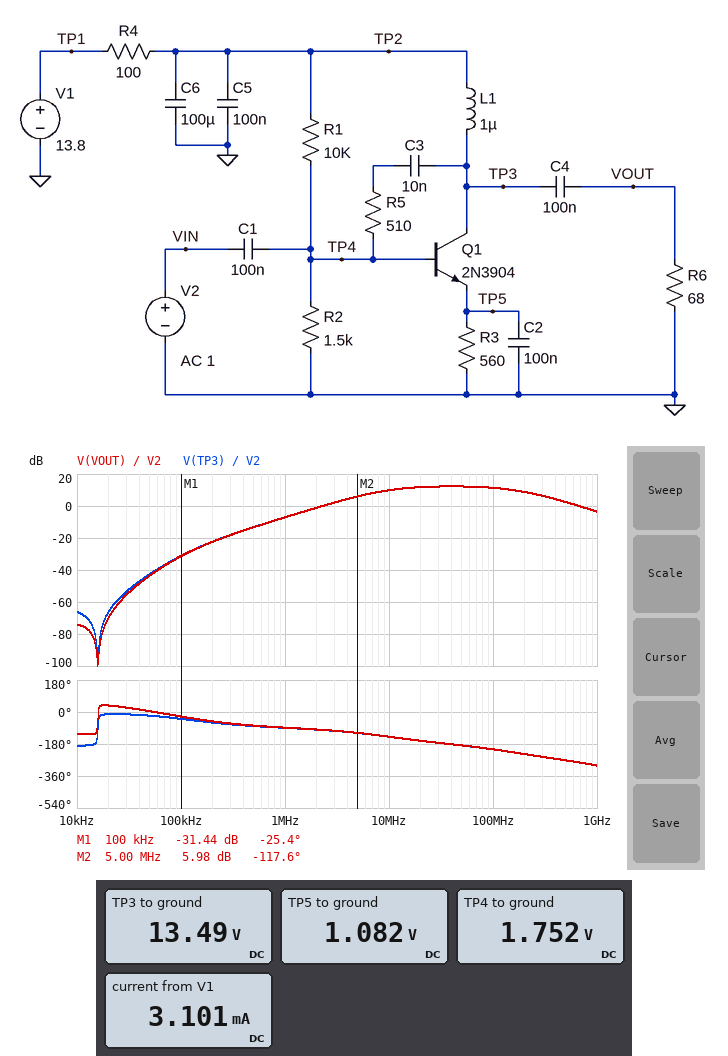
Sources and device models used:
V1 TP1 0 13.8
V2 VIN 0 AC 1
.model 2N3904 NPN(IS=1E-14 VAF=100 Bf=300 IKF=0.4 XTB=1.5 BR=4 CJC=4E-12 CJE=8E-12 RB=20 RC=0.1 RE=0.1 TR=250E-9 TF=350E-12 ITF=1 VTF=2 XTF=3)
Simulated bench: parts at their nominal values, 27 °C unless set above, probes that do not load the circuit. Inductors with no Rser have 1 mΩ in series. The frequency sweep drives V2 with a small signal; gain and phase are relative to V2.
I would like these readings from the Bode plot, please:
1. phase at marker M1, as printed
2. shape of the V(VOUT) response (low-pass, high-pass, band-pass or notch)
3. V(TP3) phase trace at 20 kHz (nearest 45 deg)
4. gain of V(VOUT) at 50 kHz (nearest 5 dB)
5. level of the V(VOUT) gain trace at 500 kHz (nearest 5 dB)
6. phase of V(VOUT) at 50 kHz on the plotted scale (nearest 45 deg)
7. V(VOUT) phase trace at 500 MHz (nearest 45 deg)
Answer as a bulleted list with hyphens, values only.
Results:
- -25.4 deg
- band-pass
- 0 deg
- -45 dB
- -15 dB
- 0 deg
- -270 deg
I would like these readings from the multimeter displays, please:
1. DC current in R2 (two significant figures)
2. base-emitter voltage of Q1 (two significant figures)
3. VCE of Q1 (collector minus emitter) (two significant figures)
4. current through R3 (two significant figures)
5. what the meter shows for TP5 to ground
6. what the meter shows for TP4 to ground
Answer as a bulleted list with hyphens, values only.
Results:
- 1.2 mA
- 670 mV
- 12 V
- 1.9 mA
- 1.082 V
- 1.752 V
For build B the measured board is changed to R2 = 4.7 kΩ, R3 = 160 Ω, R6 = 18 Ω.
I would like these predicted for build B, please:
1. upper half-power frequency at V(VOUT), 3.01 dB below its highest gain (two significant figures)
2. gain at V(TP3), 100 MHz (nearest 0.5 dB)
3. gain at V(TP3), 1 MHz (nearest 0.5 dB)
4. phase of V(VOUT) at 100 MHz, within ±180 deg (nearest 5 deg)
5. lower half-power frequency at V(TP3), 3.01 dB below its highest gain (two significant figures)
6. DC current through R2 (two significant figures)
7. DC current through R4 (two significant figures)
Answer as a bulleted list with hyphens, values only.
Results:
- 37 MHz
- 10.0 dB
- 8.5 dB
- 110 deg
- 2.6 MHz
- 770 µA
- 19 mA
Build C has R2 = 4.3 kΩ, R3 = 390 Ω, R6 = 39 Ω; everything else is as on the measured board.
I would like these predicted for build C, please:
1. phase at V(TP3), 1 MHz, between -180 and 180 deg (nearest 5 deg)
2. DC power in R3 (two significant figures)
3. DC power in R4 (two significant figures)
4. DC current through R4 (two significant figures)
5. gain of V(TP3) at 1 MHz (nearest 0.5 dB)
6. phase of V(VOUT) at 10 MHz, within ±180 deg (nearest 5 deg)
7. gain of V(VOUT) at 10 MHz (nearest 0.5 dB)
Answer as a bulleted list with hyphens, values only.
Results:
- -75 deg
- 25 mW
- 7.8 mW
- 8.8 mA
- 4.0 dB
- -155 deg
- 19.0 dB
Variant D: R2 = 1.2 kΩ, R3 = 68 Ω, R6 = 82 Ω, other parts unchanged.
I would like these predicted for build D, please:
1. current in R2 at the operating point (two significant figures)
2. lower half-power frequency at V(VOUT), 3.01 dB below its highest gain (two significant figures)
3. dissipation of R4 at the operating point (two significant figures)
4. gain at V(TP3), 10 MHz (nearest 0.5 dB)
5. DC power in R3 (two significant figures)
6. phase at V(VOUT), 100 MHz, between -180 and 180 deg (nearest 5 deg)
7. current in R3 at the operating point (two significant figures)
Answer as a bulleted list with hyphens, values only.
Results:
- 1.1 mA
- 8.3 MHz
- 11 mW
- 24.0 dB
- 5.8 mW
- 115 deg
- 9.2 mA
